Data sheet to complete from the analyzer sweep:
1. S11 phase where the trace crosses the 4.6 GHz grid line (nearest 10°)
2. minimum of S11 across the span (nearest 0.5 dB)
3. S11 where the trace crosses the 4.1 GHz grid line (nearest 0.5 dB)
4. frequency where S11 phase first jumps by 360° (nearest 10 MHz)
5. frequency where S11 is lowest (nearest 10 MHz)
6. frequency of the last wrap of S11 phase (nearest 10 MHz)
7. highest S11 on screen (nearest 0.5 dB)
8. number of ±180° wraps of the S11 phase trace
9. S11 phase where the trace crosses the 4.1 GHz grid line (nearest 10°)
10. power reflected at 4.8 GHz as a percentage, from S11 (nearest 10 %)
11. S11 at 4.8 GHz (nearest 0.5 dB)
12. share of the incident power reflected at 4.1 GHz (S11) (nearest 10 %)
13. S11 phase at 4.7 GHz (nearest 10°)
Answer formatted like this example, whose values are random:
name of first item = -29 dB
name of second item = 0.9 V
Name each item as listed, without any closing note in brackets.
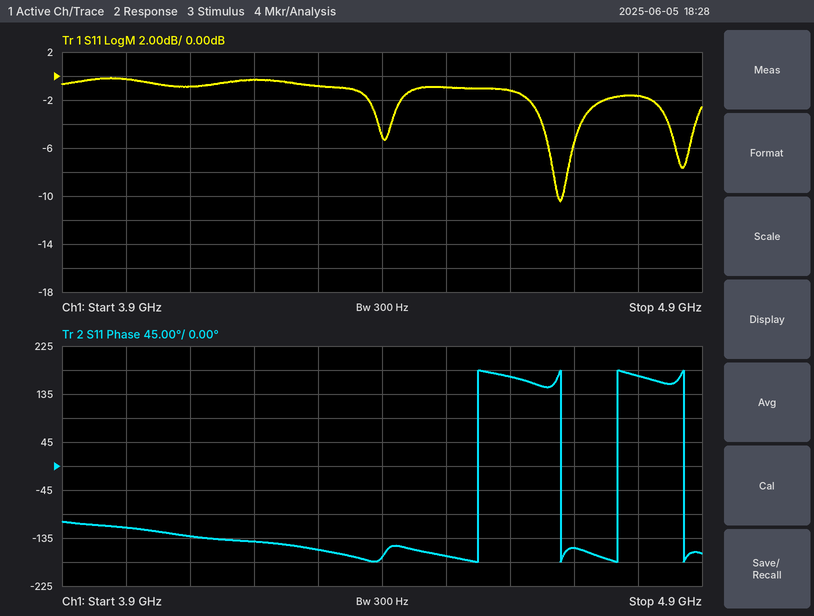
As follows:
S11 phase where the trace crosses the 4.6 GHz grid line = 170°
minimum of S11 across the span = -10.5 dB
S11 where the trace crosses the 4.1 GHz grid line = -1.0 dB
frequency where S11 phase first jumps by 360° = 4.55 GHz
frequency where S11 is lowest = 4.68 GHz
frequency of the last wrap of S11 phase = 4.87 GHz
highest S11 on screen = 0.0 dB
number of ±180° wraps of the S11 phase trace = 4
S11 phase where the trace crosses the 4.1 GHz grid line = -130°
power reflected at 4.8 GHz as a percentage, from S11 = 70 %
S11 at 4.8 GHz = -1.5 dB
share of the incident power reflected at 4.1 GHz (S11) = 80 %
S11 phase at 4.7 GHz = -150°
